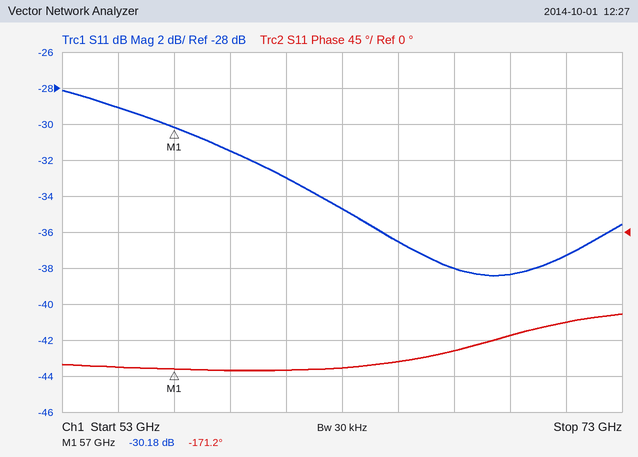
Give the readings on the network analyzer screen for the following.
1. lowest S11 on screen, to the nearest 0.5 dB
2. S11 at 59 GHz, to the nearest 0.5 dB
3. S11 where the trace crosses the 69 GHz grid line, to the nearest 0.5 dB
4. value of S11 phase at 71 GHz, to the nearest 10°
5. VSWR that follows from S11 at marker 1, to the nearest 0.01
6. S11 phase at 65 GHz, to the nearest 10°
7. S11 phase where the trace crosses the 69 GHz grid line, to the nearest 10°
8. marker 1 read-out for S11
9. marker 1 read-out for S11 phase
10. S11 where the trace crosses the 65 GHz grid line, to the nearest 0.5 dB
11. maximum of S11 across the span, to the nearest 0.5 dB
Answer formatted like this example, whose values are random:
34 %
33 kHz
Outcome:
-38.5 dB
-31.5 dB
-38.5 dB
-110°
1.06
-160°
-130°
-30.18 dB
-171.2°
-36.5 dB
-28.0 dB
